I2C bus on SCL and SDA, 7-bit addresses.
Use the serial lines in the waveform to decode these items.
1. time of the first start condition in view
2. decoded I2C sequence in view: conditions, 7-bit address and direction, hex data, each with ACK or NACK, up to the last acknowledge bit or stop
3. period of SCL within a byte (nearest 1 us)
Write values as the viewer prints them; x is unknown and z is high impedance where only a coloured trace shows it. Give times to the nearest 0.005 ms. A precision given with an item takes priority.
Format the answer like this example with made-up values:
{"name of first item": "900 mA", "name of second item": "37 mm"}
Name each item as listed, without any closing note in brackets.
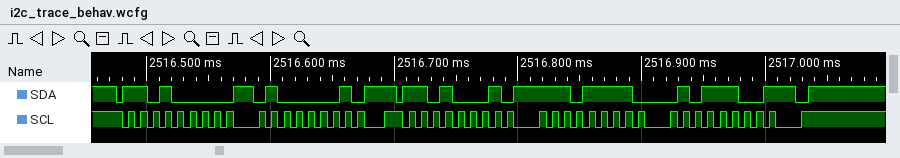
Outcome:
{"time of the first start condition in view": "2516.475 ms", "decoded I2C sequence in view: conditions, 7-bit address and direction, hex data, each with ACK or NACK, up to the last acknowledge bit or stop": "start, address 68 write ACK, 41 ACK, repeated start, address 68 read ACK, EF ACK, 5C NACK, stop", "period of SCL within a byte": "10 us"}
